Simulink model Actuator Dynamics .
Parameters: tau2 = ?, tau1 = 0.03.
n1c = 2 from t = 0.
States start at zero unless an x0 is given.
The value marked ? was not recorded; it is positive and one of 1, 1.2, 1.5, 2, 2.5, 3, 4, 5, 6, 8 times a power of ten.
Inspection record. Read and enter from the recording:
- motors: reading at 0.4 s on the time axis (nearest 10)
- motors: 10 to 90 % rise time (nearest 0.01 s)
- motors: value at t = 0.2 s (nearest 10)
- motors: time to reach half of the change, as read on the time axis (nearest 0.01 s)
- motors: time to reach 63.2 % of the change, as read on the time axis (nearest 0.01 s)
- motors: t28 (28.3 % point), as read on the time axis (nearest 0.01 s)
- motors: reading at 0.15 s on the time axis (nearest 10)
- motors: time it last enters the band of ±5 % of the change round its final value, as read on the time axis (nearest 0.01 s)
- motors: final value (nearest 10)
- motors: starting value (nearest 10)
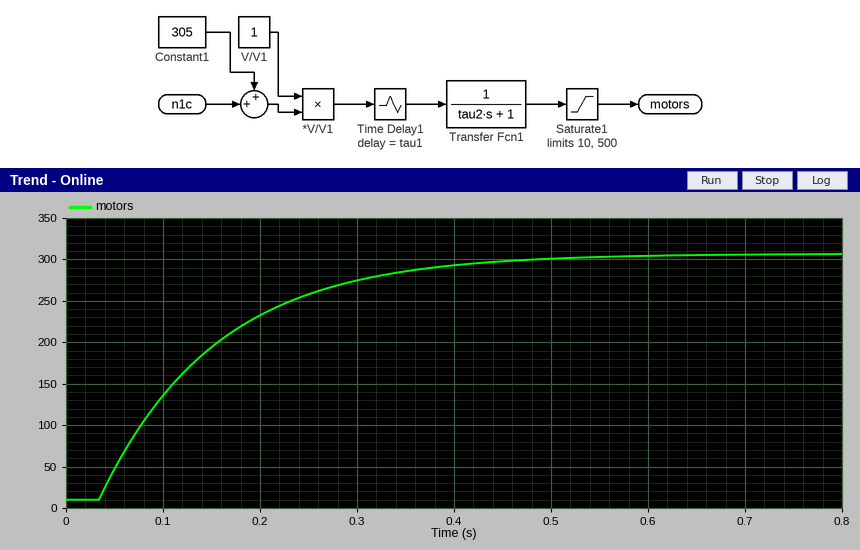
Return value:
290
0.26 s
230
0.12 s
0.15 s
0.07 s
190
0.39 s
310
10
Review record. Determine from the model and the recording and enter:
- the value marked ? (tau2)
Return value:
0.12
